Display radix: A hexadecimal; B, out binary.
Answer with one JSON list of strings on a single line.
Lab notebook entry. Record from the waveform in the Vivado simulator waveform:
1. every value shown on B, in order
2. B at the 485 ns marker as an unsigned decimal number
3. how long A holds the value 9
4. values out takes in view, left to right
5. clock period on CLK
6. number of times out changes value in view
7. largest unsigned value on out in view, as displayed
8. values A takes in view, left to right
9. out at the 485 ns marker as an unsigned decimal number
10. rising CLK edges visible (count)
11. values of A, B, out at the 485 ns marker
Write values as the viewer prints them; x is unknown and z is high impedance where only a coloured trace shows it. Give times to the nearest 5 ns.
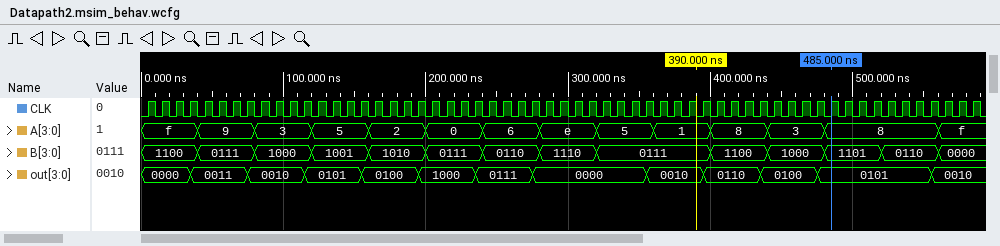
["1100, 0111, 1000, 1001, 1010, 0111, 0110, 1110, 0111, 1100, 1000, 1101, 0110, 0000", "13", "40 ns", "0000, 0011, 0010, 0101, 0100, 1000, 0111, 0000, 0010, 0110, 0100, 0101, 0010", "10 ns", "12", "1000", "f, 9, 3, 5, 2, 0, 6, e, 5, 1, 8, 3, 8, f", "5", "59", "A=8, B=1101, out=0101"]
